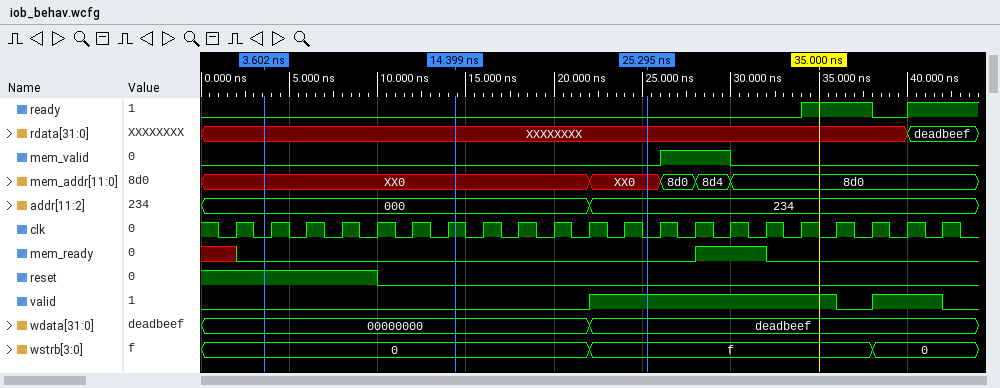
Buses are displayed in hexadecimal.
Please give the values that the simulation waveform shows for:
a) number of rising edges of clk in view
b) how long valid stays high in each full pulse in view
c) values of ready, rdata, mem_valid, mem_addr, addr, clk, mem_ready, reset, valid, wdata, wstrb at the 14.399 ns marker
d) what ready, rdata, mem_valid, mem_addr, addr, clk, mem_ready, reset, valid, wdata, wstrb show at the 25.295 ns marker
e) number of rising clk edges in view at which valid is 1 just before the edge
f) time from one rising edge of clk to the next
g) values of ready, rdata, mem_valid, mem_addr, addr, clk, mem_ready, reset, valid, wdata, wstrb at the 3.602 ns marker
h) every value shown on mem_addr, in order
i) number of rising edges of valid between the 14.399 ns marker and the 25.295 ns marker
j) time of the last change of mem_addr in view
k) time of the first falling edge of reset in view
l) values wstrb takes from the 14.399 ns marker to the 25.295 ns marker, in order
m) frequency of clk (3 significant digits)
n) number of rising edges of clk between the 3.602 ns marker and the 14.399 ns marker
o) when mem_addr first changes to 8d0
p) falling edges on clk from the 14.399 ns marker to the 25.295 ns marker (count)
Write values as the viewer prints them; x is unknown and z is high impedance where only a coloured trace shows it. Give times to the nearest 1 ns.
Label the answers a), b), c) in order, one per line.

a) 21
b) 14 ns, 4 ns
c) ready=0, rdata=XXXXXXXX, mem_valid=0, mem_addr=XX0, addr=000, clk=1, mem_ready=0, reset=0, valid=0, wdata=00000000, wstrb=0
d) ready=0, rdata=XXXXXXXX, mem_valid=0, mem_addr=XX0, addr=234, clk=0, mem_ready=0, reset=0, valid=1, wdata=deadbeef, wstrb=f
e) 9
f) 2 ns
g) ready=0, rdata=XXXXXXXX, mem_valid=0, mem_addr=XX0, addr=000, clk=0, mem_ready=0, reset=1, valid=0, wdata=00000000, wstrb=0
h) XX0, XX0, 8d0, 8d4, 8d0
i) 1
j) 30 ns
k) 10 ns
l) 0, f
m) 500 MHz
n) 6
o) 26 ns
p) 6
